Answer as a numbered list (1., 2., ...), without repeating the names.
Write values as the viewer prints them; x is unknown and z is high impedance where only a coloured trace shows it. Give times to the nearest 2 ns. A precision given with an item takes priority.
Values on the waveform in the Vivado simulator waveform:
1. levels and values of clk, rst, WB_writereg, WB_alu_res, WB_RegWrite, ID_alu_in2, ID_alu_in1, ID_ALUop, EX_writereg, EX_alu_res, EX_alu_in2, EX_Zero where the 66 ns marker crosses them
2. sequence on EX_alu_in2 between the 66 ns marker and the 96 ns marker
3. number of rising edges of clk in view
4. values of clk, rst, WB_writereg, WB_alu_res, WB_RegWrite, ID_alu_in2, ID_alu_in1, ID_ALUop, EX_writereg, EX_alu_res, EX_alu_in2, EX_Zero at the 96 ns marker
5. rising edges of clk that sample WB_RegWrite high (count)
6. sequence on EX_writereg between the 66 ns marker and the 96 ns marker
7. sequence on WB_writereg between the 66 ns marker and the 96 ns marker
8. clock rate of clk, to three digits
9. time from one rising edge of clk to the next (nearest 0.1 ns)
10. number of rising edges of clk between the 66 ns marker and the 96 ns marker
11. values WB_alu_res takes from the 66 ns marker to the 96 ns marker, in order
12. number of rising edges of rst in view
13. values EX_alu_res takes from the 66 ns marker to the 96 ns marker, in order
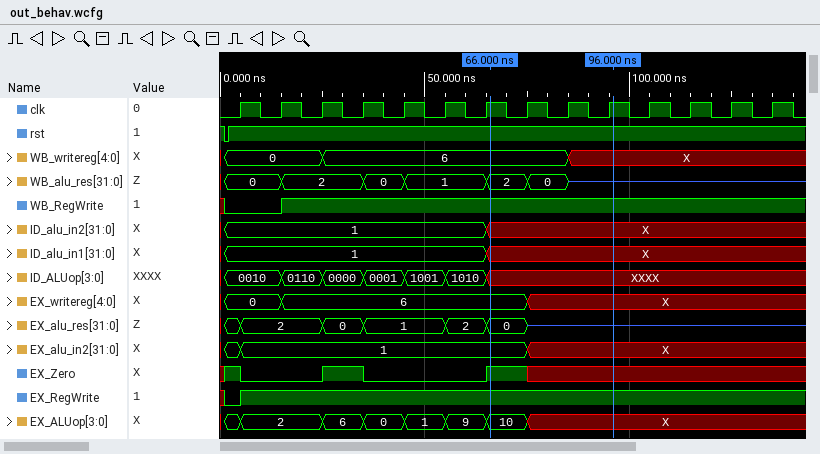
1. clk=1, rst=1, WB_writereg=6, WB_alu_res=2, WB_RegWrite=1, ID_alu_in2=X, ID_alu_in1=X, ID_ALUop=XXXX, EX_writereg=6, EX_alu_res=0, EX_alu_in2=1, EX_Zero=1
2. 1, X
3. 14
4. clk=1, rst=1, WB_writereg=X, WB_alu_res=z, WB_RegWrite=1, ID_alu_in2=X, ID_alu_in1=X, ID_ALUop=XXXX, EX_writereg=X, EX_alu_res=z, EX_alu_in2=X, EX_Zero=x
5. 12
6. 6, X
7. 6, X
8. 100 MHz
9. 10 ns
10. 3
11. 2, 0, z
12. 1
13. 0, z
